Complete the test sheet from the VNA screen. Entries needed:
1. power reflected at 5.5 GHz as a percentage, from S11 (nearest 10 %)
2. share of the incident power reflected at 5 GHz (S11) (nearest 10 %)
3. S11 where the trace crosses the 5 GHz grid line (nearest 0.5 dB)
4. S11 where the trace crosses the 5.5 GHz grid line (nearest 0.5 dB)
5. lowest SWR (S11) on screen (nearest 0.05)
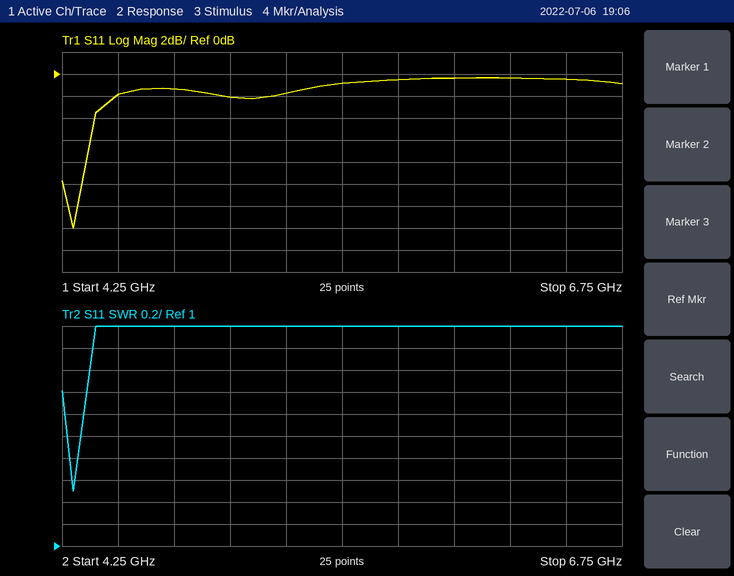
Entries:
80 %
60 %
-2.0 dB
-1.0 dB
1.50
